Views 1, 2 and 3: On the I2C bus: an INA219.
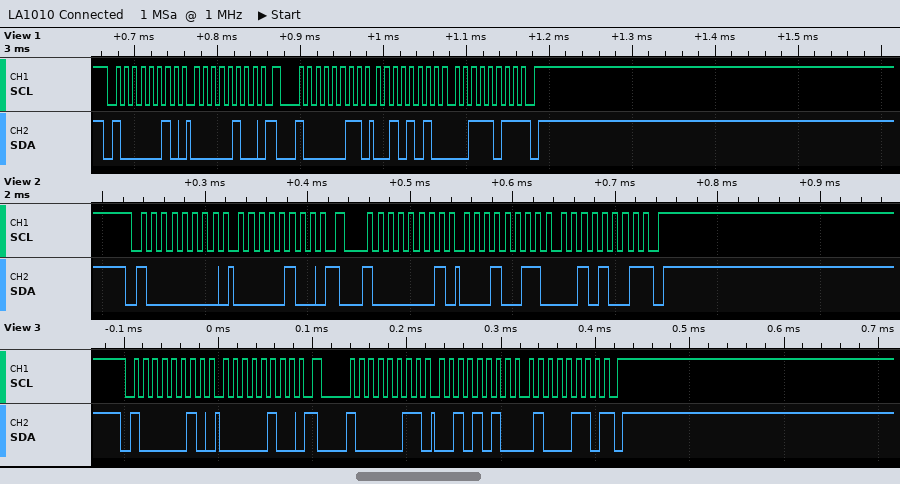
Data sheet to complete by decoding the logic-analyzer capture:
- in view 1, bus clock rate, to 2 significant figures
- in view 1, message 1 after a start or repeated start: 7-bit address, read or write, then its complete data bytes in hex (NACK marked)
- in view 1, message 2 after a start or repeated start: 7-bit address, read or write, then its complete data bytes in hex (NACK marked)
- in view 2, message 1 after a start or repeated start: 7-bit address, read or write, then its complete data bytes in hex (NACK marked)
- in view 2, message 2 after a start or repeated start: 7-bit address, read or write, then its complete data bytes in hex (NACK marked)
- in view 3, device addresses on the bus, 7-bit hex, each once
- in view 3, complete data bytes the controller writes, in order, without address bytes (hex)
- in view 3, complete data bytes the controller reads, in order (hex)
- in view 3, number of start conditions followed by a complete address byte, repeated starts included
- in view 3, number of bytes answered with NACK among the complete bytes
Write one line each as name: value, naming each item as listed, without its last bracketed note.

in view 1, bus clock rate, to 2 significant figures: 100 kHz
in view 1, message 1 after a start or repeated start: 7-bit address, read or write, then its complete data bytes in hex: 0x41 write: 04
in view 1, message 2 after a start or repeated start: 7-bit address, read or write, then its complete data bytes in hex: 0x41 read: 2A 3B NACK
in view 2, message 1 after a start or repeated start: 7-bit address, read or write, then its complete data bytes in hex: 0x40 write: 04
in view 2, message 2 after a start or repeated start: 7-bit address, read or write, then its complete data bytes in hex: 0x40 read: 13 29 NACK
in view 3, device addresses on the bus, 7-bit hex, each once: 0x41
in view 3, complete data bytes the controller writes, in order, without address bytes: 04
in view 3, complete data bytes the controller reads, in order: 2A 46
in view 3, number of start conditions followed by a complete address byte, repeated starts included: 2
in view 3, number of bytes answered with NACK among the complete bytes: 1
